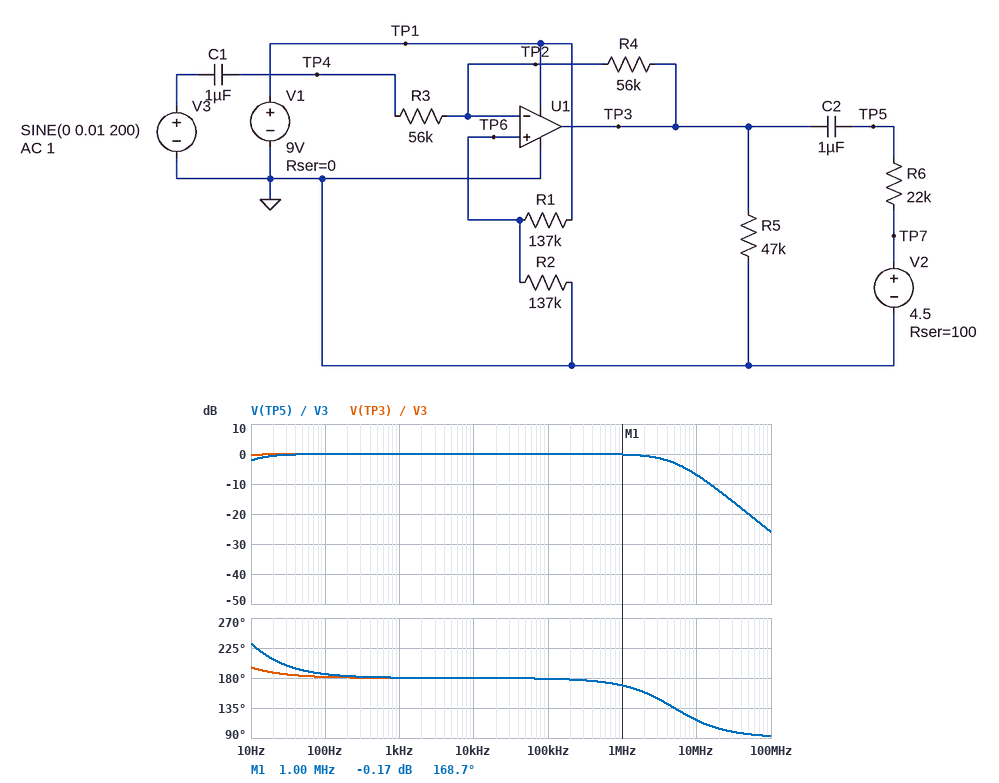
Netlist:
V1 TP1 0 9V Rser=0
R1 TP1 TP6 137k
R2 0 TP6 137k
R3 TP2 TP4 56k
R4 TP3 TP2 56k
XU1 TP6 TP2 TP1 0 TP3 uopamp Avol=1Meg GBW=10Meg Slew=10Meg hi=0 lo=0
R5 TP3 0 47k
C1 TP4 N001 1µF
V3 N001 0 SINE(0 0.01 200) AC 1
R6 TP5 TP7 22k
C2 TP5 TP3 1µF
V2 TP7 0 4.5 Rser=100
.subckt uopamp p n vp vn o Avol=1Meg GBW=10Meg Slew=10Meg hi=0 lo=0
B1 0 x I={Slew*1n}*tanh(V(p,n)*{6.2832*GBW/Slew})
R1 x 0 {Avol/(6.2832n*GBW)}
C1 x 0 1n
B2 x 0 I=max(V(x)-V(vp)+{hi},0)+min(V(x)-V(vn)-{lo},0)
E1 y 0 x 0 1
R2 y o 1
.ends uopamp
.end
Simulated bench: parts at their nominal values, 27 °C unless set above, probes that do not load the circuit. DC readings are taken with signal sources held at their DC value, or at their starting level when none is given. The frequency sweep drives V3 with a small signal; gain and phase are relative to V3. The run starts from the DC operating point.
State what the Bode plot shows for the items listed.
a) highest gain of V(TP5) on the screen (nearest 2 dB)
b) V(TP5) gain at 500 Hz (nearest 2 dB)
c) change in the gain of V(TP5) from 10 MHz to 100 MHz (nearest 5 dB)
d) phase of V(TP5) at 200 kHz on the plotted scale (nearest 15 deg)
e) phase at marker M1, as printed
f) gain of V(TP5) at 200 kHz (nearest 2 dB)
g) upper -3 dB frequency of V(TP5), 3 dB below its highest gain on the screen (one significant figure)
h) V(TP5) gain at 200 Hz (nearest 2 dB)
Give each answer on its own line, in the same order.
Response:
0 dB
0 dB
-20 dB
180 deg
168.7 deg
0 dB
5 MHz
0 dB
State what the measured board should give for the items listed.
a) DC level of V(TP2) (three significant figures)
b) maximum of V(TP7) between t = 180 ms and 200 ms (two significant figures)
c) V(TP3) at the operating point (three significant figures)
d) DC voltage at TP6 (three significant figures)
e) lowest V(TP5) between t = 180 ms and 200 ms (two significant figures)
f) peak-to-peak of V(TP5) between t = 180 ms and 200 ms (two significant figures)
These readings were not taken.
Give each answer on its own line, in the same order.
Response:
4.50 V
4.5 V
4.50 V
4.50 V
4.5 V
20 mV
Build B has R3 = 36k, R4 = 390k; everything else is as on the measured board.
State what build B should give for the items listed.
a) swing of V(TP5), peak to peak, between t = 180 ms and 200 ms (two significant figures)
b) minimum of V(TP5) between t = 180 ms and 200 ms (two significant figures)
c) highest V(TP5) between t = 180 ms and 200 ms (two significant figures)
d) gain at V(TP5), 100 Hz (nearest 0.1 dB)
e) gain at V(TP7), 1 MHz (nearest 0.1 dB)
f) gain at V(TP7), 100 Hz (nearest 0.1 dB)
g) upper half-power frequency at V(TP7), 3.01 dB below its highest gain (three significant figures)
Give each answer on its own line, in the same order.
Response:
220 mV
4.4 V
4.6 V
20.7 dB
-30.0 dB
-26.2 dB
845 kHz
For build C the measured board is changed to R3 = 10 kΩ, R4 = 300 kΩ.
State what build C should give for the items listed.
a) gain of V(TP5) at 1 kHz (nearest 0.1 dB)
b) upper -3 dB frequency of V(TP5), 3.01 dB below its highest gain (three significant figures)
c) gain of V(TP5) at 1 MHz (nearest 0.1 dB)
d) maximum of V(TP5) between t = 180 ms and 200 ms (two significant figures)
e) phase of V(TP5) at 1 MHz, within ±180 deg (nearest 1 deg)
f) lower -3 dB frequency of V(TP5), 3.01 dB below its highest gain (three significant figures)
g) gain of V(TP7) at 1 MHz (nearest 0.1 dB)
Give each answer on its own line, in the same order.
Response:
29.5 dB
323 kHz
19.3 dB
4.8 V
108 deg
18.5 Hz
-27.6 dB
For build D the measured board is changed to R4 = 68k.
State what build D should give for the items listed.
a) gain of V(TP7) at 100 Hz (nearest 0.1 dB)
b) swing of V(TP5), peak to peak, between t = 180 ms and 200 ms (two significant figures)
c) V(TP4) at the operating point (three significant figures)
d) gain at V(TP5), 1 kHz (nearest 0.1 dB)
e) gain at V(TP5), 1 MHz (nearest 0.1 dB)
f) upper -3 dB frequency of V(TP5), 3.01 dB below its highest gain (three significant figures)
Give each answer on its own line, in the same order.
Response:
-45.2 dB
24 mV
4.50 V
1.7 dB
1.5 dB
4.52 MHz
